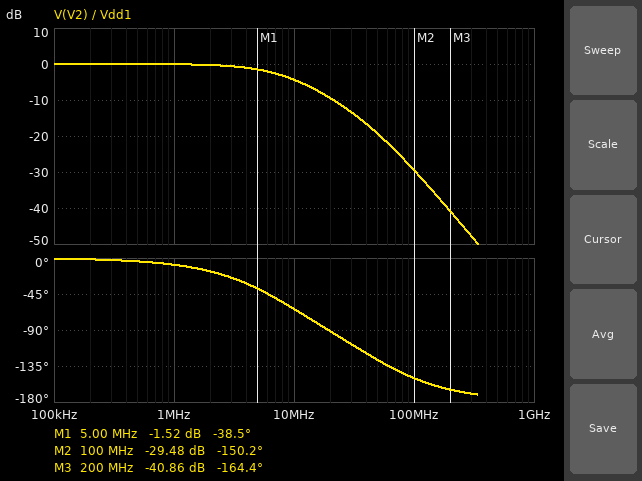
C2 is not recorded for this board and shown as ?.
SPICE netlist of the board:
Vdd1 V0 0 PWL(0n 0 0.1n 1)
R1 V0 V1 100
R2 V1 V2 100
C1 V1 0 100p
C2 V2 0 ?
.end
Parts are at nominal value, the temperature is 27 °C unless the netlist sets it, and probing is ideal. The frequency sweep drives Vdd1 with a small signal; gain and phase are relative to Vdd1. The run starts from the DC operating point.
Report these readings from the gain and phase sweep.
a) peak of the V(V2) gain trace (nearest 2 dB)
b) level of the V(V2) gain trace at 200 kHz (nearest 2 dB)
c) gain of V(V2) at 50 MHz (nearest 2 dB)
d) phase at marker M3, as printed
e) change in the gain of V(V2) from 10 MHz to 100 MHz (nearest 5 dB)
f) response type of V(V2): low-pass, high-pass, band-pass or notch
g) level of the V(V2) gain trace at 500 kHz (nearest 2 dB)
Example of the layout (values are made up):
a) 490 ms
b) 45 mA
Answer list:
a) 0 dB
b) 0 dB
c) -20 dB
d) -164.4 deg
e) -25 dB
f) low-pass
g) 0 dB
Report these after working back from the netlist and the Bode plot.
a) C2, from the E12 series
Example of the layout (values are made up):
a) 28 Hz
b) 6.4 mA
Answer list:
a) 68 pF
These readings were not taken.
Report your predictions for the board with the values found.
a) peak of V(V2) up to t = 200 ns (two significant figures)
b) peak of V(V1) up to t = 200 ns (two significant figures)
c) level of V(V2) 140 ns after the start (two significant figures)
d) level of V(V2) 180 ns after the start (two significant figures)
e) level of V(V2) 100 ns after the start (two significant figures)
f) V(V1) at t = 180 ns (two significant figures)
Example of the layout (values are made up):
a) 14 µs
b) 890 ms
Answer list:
a) 1.0 V
b) 1.0 V
c) 1.0 V
d) 1.0 V
e) 990 mV
f) 1.0 V
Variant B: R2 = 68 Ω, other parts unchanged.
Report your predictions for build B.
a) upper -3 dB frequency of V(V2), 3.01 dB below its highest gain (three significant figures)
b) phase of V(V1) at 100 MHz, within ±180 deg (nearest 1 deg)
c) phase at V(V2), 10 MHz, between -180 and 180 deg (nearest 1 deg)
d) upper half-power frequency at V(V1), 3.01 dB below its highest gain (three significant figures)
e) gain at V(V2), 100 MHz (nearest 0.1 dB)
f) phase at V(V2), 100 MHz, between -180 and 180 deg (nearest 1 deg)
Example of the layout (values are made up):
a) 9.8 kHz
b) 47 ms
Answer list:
a) 8.25 MHz
b) -71 deg
c) -59 deg
d) 8.76 MHz
e) -26.8 dB
f) -142 deg
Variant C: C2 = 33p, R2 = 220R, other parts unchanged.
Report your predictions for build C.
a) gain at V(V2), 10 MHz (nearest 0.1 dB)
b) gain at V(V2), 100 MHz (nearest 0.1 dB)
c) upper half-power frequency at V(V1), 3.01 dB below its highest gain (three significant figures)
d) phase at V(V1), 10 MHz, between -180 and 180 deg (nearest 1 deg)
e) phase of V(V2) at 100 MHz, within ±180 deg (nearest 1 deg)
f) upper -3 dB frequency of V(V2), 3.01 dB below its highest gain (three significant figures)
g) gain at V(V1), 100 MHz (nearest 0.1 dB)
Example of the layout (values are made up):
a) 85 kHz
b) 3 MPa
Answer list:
a) -3.4 dB
b) -29.7 dB
c) 11.3 MHz
d) -37 deg
e) -155 deg
f) 9.26 MHz
g) -16.3 dB
